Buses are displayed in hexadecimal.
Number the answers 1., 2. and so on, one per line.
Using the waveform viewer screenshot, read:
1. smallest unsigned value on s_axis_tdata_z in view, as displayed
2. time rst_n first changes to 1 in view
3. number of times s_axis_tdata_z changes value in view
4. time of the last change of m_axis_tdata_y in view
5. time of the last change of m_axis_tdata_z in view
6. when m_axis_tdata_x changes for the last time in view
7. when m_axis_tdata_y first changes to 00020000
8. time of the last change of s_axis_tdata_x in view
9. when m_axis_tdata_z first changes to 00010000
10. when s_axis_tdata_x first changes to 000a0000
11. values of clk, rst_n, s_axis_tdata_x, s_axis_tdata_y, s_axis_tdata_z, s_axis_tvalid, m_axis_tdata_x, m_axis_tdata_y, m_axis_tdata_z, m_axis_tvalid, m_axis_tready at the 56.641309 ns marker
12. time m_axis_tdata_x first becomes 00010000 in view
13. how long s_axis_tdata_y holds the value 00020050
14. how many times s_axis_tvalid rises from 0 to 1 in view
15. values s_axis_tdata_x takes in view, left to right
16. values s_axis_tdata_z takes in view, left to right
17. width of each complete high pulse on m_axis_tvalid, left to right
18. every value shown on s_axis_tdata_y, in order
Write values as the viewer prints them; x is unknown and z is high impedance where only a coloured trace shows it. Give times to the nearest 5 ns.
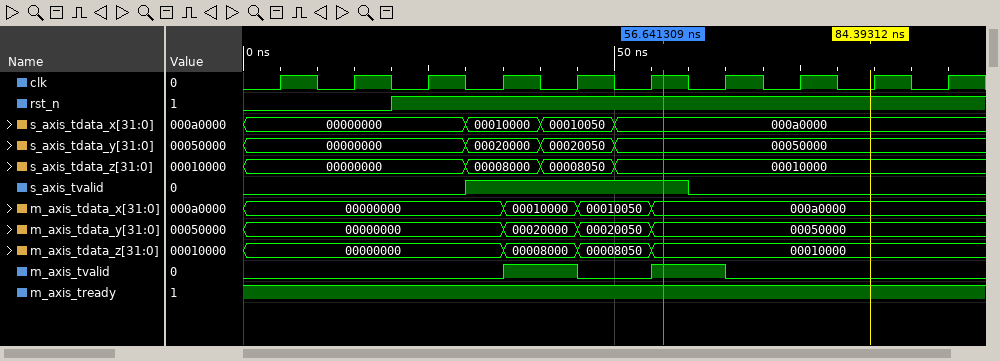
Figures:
1. 00000000
2. 20 ns
3. 3
4. 55 ns
5. 55 ns
6. 55 ns
7. 35 ns
8. 50 ns
9. 55 ns
10. 50 ns
11. clk=1, rst_n=1, s_axis_tdata_x=000a0000, s_axis_tdata_y=00050000, s_axis_tdata_z=00010000, s_axis_tvalid=1, m_axis_tdata_x=000a0000, m_axis_tdata_y=00050000, m_axis_tdata_z=00010000, m_axis_tvalid=1, m_axis_tready=1
12. 35 ns
13. 10 ns
14. 1
15. 00000000, 00010000, 00010050, 000a0000
16. 00000000, 00008000, 00008050, 00010000
17. 10 ns, 10 ns
18. 00000000, 00020000, 00020050, 00050000
